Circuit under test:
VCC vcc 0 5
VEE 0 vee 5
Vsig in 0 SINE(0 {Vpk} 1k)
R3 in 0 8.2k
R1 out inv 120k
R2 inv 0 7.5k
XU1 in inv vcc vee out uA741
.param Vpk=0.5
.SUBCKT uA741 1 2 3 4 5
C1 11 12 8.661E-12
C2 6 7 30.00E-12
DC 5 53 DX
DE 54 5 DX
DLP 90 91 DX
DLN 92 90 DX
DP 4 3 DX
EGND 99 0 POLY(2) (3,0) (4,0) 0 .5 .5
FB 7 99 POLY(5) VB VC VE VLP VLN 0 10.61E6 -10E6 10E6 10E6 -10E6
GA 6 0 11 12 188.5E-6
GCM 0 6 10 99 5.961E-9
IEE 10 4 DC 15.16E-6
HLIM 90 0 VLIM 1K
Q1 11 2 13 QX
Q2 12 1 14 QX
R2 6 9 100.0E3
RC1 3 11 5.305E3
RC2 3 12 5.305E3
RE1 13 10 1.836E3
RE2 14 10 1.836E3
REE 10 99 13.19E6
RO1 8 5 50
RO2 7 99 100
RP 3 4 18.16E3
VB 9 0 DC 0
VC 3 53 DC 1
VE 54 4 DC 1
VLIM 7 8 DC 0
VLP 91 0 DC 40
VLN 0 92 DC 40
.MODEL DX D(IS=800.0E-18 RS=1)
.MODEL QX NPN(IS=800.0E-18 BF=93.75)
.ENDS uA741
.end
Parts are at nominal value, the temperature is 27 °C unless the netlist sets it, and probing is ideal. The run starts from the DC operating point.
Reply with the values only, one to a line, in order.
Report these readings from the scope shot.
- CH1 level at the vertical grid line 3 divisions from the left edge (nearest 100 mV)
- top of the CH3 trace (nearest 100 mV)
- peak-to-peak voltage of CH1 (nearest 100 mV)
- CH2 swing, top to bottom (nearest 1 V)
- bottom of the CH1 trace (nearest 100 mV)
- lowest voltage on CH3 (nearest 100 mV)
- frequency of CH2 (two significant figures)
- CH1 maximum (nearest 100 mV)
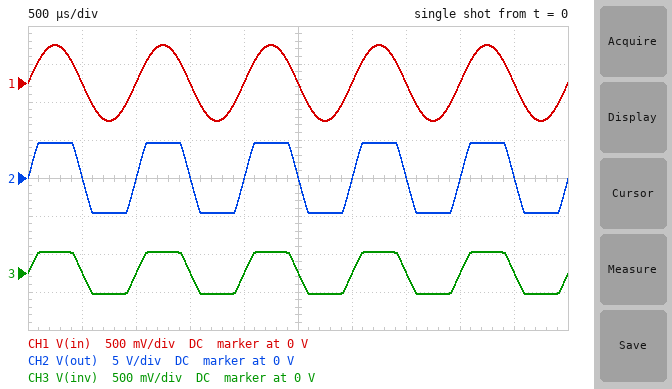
0 V
300 mV
1.0 V
9 V
-500 mV
-300 mV
1.0 kHz
500 mV
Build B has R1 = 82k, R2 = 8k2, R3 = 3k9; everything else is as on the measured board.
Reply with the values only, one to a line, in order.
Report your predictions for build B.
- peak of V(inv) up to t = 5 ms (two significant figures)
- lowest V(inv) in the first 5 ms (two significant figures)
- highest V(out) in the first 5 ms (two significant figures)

420 mV
-420 mV
4.6 V
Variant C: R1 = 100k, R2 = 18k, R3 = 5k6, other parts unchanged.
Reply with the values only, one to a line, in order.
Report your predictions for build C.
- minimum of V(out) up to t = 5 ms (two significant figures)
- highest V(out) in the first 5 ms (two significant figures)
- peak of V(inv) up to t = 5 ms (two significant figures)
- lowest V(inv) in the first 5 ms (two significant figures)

-3.3 V
3.3 V
500 mV
-500 mV
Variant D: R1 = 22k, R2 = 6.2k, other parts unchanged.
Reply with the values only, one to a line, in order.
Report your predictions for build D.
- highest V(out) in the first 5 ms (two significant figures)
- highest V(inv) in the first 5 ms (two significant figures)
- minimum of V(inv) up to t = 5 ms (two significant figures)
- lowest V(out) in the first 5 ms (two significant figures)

2.3 V
500 mV
-500 mV
-2.3 V
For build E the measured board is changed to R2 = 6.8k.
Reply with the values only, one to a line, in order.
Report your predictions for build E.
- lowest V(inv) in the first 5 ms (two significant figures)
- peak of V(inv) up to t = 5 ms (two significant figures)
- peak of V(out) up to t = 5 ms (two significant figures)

-250 mV
250 mV
4.6 V
